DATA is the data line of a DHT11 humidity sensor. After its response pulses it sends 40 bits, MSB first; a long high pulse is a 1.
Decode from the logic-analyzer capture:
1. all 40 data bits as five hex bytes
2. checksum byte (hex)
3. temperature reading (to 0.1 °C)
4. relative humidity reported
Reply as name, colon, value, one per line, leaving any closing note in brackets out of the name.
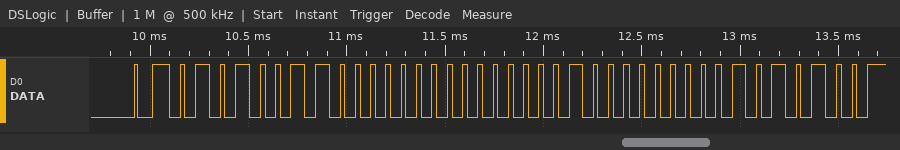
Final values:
all 40 data bits as five hex bytes: 53 00 01 00 54
checksum byte: 0x54
temperature reading: 1.0 °C
relative humidity reported: 83 %
